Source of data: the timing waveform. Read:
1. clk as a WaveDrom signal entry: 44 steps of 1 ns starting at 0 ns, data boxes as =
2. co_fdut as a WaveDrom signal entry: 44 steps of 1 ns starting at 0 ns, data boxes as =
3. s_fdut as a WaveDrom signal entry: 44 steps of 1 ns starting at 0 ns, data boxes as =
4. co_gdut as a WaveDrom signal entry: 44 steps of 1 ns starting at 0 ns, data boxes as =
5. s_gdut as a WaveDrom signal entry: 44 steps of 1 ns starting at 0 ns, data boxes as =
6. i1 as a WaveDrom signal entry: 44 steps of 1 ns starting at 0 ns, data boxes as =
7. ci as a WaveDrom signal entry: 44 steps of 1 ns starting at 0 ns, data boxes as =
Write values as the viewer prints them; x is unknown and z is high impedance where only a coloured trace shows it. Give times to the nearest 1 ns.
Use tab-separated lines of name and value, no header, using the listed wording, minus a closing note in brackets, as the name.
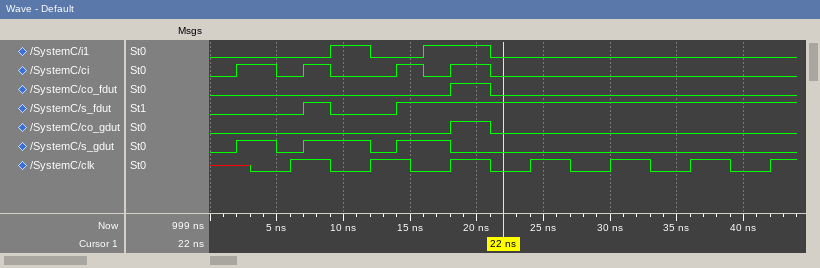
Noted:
clk as a WaveDrom signal entry: 44 steps of 1 ns starting at 0 ns, data boxes as =	{name: 'clk', wave: 'x..0..1..0..1..0..1..0..1..0..1..0..1..0..1.'}
co_fdut as a WaveDrom signal entry: 44 steps of 1 ns starting at 0 ns, data boxes as =	{name: 'co_fdut', wave: '0.................1..0......................'}
s_fdut as a WaveDrom signal entry: 44 steps of 1 ns starting at 0 ns, data boxes as =	{name: 's_fdut', wave: '0......1.0....1.............................'}
co_gdut as a WaveDrom signal entry: 44 steps of 1 ns starting at 0 ns, data boxes as =	{name: 'co_gdut', wave: '0.................1..0......................'}
s_gdut as a WaveDrom signal entry: 44 steps of 1 ns starting at 0 ns, data boxes as =	{name: 's_gdut', wave: '0.1..0.1....0.1...0.........................'}
i1 as a WaveDrom signal entry: 44 steps of 1 ns starting at 0 ns, data boxes as =	{name: 'i1', wave: '0........1..0...1....0......................'}
ci as a WaveDrom signal entry: 44 steps of 1 ns starting at 0 ns, data boxes as =	{name: 'ci', wave: '0.1..0.1.0....1.0.1..0......................'}
